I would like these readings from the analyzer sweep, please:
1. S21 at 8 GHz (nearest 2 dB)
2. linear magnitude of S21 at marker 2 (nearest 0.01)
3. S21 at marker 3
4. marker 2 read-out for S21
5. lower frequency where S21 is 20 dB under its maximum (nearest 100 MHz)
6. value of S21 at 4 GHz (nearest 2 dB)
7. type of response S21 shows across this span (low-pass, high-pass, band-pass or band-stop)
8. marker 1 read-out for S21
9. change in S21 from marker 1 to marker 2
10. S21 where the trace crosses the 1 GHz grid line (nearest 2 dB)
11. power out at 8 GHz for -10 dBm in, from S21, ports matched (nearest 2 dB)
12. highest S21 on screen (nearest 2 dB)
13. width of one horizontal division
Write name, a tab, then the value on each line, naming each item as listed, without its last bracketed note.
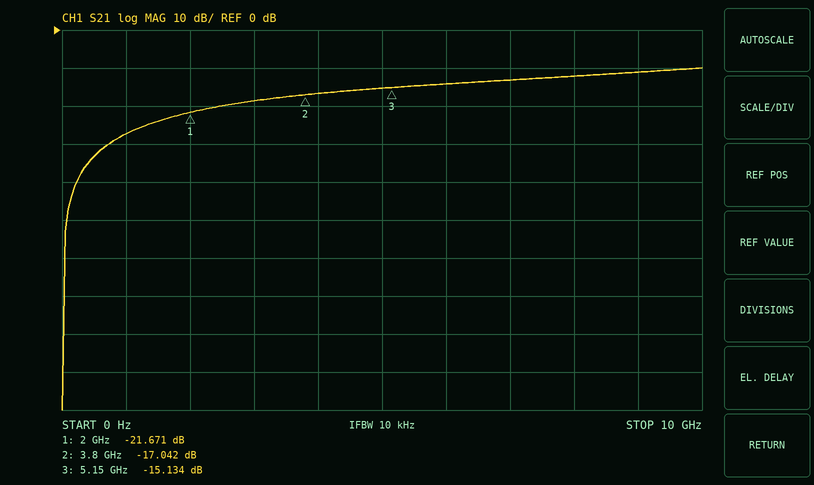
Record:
S21 at 8 GHz	-12 dB
linear magnitude of S21 at marker 2	0.14
S21 at marker 3	-15.134 dB
marker 2 read-out for S21	-17.042 dB
lower frequency where S21 is 20 dB under its maximum	700 MHz
value of S21 at 4 GHz	-16 dB
type of response S21 shows across this span	high-pass
marker 1 read-out for S21	-21.671 dB
change in S21 from marker 1 to marker 2	4.629 dB
S21 where the trace crosses the 1 GHz grid line	-28 dB
power out at 8 GHz for -10 dBm in, from S21, ports matched	-22 dBm
highest S21 on screen	-10 dB
width of one horizontal division	1 GHz
